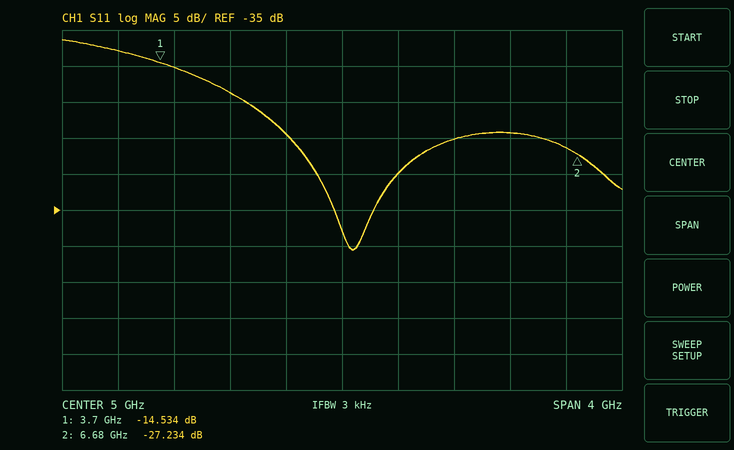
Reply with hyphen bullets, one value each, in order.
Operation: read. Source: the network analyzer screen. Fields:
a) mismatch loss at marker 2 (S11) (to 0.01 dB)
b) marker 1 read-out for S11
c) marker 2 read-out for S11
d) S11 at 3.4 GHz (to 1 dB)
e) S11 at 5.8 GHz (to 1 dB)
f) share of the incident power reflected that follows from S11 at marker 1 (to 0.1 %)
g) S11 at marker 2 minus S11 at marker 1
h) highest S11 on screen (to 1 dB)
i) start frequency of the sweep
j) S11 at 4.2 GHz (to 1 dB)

- 0.01 dB
- -14.534 dB
- -27.234 dB
- -13 dB
- -25 dB
- 3.5 %
- -12.700 dB
- -11 dB
- 3 GHz
- -19 dB
